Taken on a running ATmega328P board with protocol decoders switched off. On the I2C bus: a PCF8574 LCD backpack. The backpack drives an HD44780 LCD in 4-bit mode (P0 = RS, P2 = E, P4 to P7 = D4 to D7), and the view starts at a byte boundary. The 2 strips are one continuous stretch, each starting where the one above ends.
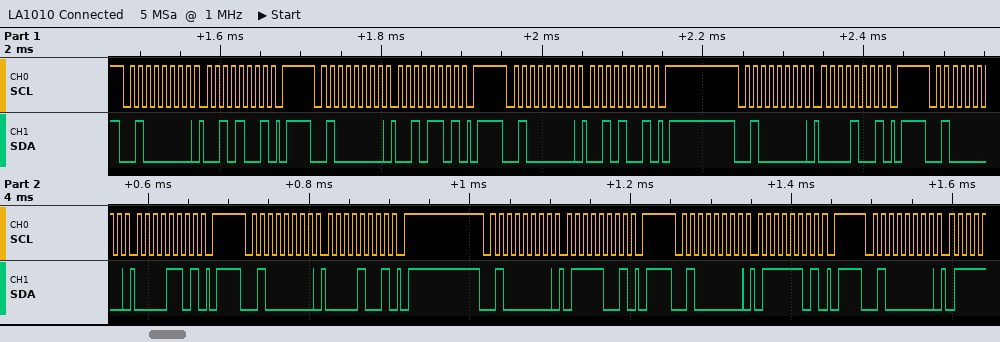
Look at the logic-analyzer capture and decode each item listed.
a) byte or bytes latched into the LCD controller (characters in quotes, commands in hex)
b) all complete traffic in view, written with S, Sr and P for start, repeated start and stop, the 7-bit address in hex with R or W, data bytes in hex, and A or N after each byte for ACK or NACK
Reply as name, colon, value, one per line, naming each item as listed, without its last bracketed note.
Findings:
byte or bytes latched into the LCD controller: ' '
all complete traffic in view, written with S, Sr and P for start, repeated start and stop, the 7-bit address in hex with R or W, data bytes in hex, and A or N after each byte for ACK or NACK: S 20W A 29 A P S 20W A 2D A P S 20W A 29 A P S 20W A 09 A P S 20W A 0D A P S 20W A 09 A P S 20W A 79 A P S 20W A 7D A P S 20W A
